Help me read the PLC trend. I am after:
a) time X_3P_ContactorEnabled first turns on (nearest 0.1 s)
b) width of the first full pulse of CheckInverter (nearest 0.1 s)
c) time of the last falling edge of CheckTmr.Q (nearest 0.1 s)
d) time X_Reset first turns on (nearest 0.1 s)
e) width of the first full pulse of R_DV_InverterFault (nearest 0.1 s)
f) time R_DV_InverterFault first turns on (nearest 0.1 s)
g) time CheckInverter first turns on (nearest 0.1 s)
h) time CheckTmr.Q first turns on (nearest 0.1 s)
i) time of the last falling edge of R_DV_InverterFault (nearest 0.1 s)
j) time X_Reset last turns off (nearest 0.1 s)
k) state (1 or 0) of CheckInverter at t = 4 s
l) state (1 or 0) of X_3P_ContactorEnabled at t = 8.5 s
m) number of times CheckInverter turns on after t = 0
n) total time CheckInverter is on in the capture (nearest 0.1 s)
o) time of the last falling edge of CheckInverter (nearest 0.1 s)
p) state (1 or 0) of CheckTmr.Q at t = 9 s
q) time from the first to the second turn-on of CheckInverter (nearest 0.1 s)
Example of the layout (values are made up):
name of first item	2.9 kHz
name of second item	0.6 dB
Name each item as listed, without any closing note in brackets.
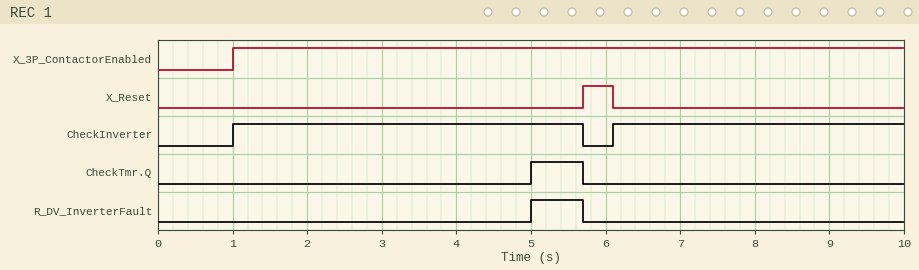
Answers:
time X_3P_ContactorEnabled first turns on	1.0 s
width of the first full pulse of CheckInverter	4.7 s
time of the last falling edge of CheckTmr.Q	5.7 s
time X_Reset first turns on	5.7 s
width of the first full pulse of R_DV_InverterFault	0.7 s
time R_DV_InverterFault first turns on	5.0 s
time CheckInverter first turns on	1.0 s
time CheckTmr.Q first turns on	5.0 s
time of the last falling edge of R_DV_InverterFault	5.7 s
time X_Reset last turns off	6.1 s
state (1 or 0) of CheckInverter at t = 4 s	1
state (1 or 0) of X_3P_ContactorEnabled at t = 8.5 s	1
number of times CheckInverter turns on after t = 0	2
total time CheckInverter is on in the capture	8.6 s
time of the last falling edge of CheckInverter	5.7 s
state (1 or 0) of CheckTmr.Q at t = 9 s	0
time from the first to the second turn-on of CheckInverter	5.1 s
